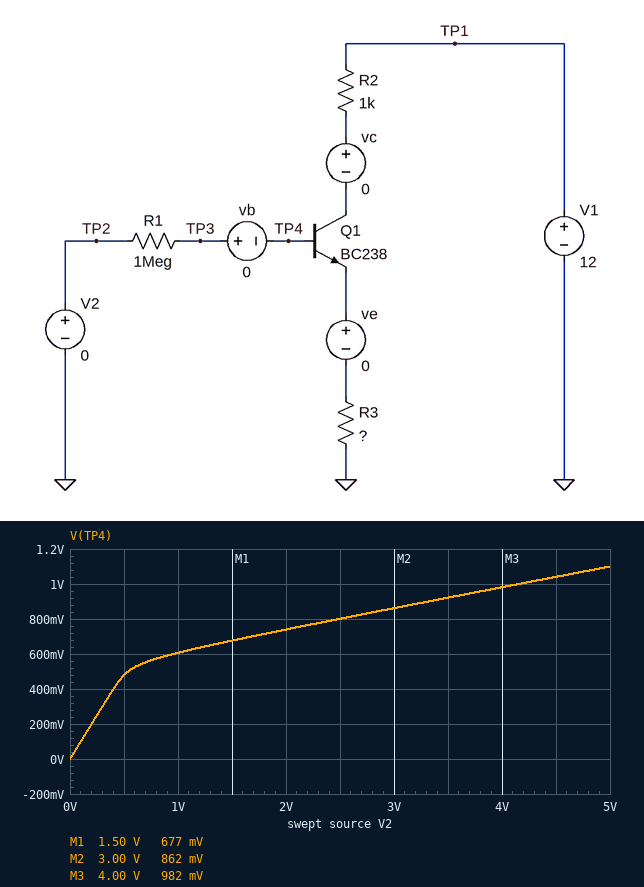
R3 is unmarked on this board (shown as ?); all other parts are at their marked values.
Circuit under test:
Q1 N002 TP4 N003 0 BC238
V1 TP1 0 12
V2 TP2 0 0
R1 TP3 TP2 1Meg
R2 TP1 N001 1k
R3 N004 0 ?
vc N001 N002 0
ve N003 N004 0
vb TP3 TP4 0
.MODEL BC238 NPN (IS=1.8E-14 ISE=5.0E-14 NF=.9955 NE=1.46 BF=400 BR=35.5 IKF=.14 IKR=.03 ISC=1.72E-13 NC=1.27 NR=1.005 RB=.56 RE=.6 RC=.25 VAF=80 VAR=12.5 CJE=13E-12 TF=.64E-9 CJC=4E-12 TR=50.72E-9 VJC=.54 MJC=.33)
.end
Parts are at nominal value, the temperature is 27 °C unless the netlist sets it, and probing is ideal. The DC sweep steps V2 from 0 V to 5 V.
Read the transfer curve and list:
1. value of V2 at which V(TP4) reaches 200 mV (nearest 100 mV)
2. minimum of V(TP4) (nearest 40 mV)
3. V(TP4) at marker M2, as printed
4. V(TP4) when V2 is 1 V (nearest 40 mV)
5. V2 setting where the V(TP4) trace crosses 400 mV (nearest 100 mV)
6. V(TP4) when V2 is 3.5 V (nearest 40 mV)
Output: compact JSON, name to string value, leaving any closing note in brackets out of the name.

{"value of V2 at which V(TP4) reaches 200 mV": "200 mV", "minimum of V(TP4)": "0 V", "V(TP4) at marker M2, as printed": "862 mV", "V(TP4) when V2 is 1 V": "600 mV", "V2 setting where the V(TP4) trace crosses 400 mV": "400 mV", "V(TP4) when V2 is 3.5 V": "920 mV"}
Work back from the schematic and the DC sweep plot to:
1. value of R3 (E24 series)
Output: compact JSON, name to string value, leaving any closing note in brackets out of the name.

{"value of R3": "390 Ω"}
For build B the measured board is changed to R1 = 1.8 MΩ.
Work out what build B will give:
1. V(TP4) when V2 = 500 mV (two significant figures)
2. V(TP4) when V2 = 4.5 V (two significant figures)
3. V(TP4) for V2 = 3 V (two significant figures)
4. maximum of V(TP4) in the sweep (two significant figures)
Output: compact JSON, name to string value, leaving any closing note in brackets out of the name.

{"V(TP4) when V2 = 500 mV": "470 mV", "V(TP4) when V2 = 4.5 V": "850 mV", "V(TP4) for V2 = 3 V": "740 mV", "maximum of V(TP4) in the sweep": "880 mV"}
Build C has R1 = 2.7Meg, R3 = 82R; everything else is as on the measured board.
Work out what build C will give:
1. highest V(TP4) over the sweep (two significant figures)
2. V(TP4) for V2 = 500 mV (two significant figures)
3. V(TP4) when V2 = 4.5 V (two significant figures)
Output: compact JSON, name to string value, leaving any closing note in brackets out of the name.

{"highest V(TP4) over the sweep": "650 mV", "V(TP4) for V2 = 500 mV": "460 mV", "V(TP4) when V2 = 4.5 V": "640 mV"}
